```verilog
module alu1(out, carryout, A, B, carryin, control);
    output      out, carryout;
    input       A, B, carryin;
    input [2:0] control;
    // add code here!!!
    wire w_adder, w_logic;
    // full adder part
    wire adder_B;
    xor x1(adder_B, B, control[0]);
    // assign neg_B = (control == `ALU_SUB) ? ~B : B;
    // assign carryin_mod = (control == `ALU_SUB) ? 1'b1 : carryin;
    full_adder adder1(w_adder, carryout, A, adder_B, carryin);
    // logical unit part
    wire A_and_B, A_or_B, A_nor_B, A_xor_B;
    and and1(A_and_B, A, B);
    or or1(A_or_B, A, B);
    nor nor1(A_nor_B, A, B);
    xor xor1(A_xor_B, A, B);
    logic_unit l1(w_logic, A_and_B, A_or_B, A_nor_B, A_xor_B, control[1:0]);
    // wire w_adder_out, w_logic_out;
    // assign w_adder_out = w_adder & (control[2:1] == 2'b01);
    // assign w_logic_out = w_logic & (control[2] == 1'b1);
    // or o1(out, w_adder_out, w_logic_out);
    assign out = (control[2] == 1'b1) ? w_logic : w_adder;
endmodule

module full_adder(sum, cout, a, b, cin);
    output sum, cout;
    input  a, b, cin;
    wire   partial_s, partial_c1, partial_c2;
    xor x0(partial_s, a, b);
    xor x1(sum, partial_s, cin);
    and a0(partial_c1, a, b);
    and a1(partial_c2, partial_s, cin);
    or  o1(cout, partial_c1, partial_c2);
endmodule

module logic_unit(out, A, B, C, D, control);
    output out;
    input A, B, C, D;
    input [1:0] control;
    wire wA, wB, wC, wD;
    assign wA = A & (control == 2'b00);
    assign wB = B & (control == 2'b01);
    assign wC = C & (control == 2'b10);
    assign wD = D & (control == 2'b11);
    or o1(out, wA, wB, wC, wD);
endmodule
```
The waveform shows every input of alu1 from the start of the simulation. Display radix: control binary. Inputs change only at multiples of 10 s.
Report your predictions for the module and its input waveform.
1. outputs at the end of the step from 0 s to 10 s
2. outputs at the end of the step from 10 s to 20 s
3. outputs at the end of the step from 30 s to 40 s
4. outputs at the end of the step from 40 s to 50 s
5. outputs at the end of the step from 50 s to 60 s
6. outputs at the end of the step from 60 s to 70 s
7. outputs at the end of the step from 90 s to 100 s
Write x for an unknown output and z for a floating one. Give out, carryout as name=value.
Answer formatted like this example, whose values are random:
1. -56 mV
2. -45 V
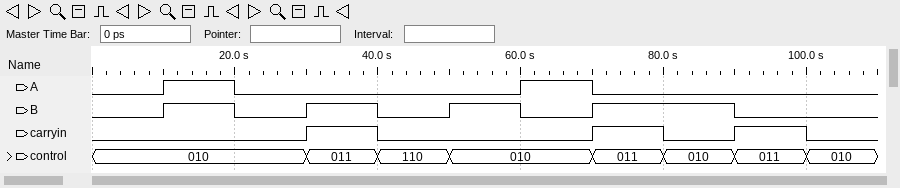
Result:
1. out=0, carryout=0
2. out=0, carryout=1
3. out=1, carryout=0
4. out=1, carryout=0
5. out=1, carryout=0
6. out=1, carryout=0
7. out=0, carryout=1
